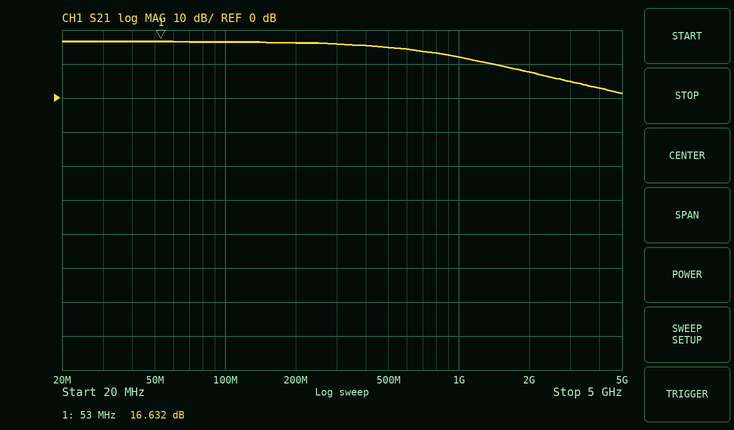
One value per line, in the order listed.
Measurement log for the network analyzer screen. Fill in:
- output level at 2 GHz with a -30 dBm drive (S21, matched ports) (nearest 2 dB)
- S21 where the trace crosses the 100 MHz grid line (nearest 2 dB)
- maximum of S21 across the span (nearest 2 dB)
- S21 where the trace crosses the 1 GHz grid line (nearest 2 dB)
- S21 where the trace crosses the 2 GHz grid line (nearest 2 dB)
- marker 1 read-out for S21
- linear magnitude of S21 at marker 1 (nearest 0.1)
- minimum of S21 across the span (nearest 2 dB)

-22 dBm
16 dB
16 dB
12 dB
8 dB
16.632 dB
6.8
2 dB
